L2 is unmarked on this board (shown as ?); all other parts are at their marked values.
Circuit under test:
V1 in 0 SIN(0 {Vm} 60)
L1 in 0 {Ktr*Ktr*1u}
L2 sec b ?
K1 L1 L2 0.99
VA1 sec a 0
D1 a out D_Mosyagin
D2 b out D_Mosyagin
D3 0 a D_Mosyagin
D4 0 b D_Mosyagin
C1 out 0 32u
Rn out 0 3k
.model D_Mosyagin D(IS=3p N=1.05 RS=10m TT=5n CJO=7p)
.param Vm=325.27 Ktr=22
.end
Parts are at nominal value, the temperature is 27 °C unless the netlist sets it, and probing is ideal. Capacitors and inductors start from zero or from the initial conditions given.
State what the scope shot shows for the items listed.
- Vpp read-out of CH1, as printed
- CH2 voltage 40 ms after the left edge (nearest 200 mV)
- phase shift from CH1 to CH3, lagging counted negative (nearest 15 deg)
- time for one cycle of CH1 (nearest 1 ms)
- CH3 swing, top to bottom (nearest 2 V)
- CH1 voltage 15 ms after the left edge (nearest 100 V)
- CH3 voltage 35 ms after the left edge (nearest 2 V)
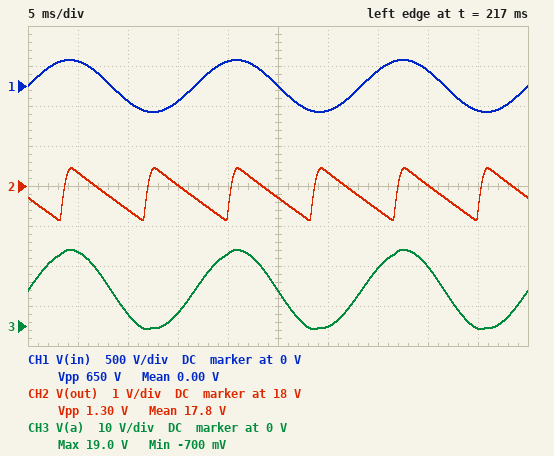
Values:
650 V
18.0 V
0 deg
17 ms
20 V
-200 V
14 V
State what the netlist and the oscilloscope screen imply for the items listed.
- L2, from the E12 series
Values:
1.8 µH
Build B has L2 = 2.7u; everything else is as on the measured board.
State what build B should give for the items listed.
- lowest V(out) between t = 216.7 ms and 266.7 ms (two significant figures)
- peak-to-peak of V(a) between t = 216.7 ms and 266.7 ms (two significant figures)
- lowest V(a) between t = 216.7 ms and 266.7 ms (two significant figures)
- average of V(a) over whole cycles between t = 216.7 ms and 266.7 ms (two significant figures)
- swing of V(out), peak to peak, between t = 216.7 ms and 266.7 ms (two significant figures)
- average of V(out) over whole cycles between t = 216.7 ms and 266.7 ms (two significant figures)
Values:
21 V
24 V
-660 mV
11 V
1.6 V
22 V
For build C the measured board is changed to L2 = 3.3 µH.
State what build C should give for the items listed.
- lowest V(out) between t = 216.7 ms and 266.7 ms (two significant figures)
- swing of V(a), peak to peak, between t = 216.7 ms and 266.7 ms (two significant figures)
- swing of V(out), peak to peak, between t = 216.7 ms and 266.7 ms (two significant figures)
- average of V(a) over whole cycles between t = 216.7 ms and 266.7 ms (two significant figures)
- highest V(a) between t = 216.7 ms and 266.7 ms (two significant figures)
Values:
24 V
27 V
1.8 V
12 V
26 V
